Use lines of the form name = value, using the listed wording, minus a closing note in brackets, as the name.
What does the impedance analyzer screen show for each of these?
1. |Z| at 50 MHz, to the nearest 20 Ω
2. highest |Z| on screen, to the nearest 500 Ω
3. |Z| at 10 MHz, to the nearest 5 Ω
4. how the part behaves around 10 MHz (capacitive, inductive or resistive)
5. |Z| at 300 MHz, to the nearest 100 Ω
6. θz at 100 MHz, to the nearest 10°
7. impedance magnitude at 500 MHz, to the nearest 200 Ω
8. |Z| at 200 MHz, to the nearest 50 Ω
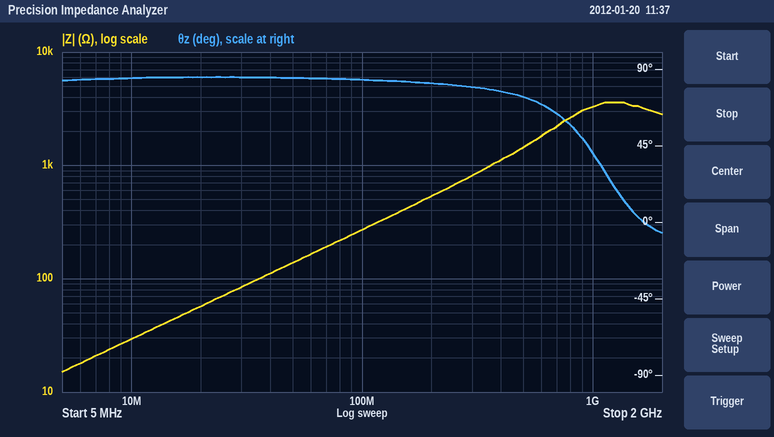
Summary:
|Z| at 50 MHz, to the nearest 20 Ω = 140 Ω
highest |Z| on screen, to the nearest 500 Ω = 3.5 kΩ
|Z| at 10 MHz, to the nearest 5 Ω = 30 Ω
how the part behaves around 10 MHz = inductive
|Z| at 300 MHz, to the nearest 100 Ω = 800 Ω
θz at 100 MHz, to the nearest 10° = 80°
impedance magnitude at 500 MHz, to the nearest 200 Ω = 1.4 kΩ
|Z| at 200 MHz, to the nearest 50 Ω = 550 Ω
